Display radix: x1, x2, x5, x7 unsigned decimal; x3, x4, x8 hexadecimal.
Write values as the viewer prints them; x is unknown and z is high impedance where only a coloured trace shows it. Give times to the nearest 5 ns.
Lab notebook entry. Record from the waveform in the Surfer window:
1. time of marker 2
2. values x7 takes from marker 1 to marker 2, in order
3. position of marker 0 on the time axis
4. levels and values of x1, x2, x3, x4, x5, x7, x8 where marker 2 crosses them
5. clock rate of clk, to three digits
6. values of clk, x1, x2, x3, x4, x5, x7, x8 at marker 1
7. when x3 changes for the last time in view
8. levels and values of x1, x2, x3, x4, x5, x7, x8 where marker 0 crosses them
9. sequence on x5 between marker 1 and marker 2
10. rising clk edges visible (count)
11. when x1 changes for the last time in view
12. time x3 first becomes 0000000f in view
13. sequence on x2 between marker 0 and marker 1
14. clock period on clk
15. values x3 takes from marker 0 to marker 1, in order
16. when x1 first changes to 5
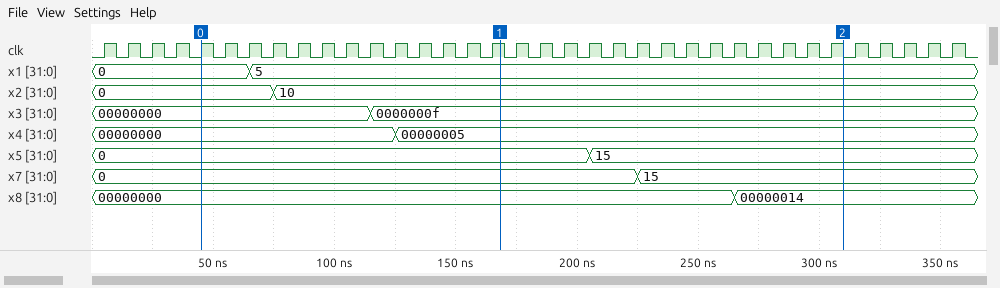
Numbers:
310 ns
0, 15
45 ns
x1=5, x2=10, x3=0000000f, x4=00000005, x5=15, x7=15, x8=00000014
100 MHz
clk=1, x1=5, x2=10, x3=0000000f, x4=00000005, x5=0, x7=0, x8=00000000
115 ns
x1=0, x2=0, x3=00000000, x4=00000000, x5=0, x7=0, x8=00000000
0, 15
36
65 ns
115 ns
0, 10
10 ns
00000000, 0000000f
65 ns
